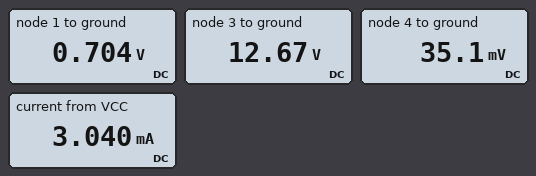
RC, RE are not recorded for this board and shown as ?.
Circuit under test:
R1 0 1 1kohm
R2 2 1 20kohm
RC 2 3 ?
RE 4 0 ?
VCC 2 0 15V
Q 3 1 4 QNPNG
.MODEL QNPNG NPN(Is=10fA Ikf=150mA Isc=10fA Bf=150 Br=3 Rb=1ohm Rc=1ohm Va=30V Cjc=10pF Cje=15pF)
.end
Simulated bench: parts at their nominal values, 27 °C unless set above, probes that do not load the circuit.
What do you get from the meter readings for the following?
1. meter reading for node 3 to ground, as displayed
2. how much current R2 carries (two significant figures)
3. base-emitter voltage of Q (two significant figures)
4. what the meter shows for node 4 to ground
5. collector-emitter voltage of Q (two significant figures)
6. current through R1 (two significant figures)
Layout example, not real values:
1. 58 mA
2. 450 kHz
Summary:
1. 12.67 V
2. 710 µA
3. 670 mV
4. 35.1 mV
5. 13 V
6. 700 µA
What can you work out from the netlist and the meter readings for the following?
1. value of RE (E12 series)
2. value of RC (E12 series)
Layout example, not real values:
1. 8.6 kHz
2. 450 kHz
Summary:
1. 15 Ω
2. 1 kΩ
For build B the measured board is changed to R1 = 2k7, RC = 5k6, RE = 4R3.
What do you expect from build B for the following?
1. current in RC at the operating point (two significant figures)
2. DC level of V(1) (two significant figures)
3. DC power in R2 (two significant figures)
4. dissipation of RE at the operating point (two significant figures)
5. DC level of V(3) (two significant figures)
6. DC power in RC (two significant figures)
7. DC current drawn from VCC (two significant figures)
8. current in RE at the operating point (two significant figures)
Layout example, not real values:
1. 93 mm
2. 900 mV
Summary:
1. 2.7 mA
2. 710 mV
3. 10 mW
4. 42 µW
5. 49 mV
6. 40 mW
7. 3.4 mA
8. 3.1 mA
